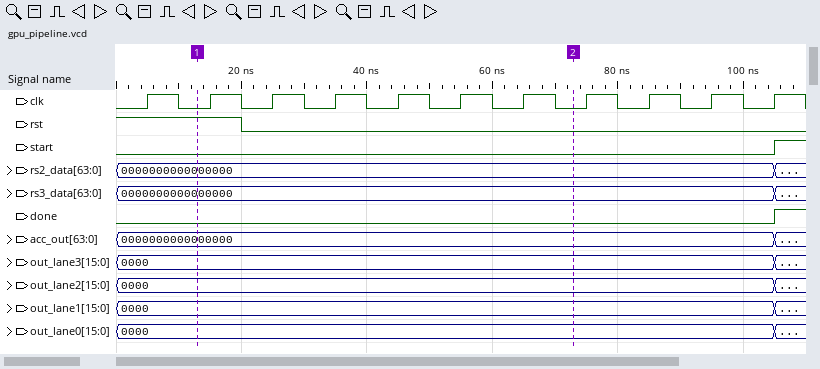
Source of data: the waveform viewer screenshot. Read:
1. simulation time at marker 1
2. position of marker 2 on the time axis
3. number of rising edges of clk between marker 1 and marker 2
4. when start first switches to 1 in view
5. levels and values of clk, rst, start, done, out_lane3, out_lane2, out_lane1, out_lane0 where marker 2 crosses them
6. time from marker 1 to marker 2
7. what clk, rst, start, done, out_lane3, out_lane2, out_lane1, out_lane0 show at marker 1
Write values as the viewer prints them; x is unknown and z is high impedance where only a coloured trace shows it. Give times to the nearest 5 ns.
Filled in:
15 ns
75 ns
6
105 ns
clk=0, rst=0, start=0, done=0, out_lane3=0000, out_lane2=0000, out_lane1=0000, out_lane0=0000
60 ns
clk=0, rst=1, start=0, done=0, out_lane3=0000, out_lane2=0000, out_lane1=0000, out_lane0=0000
